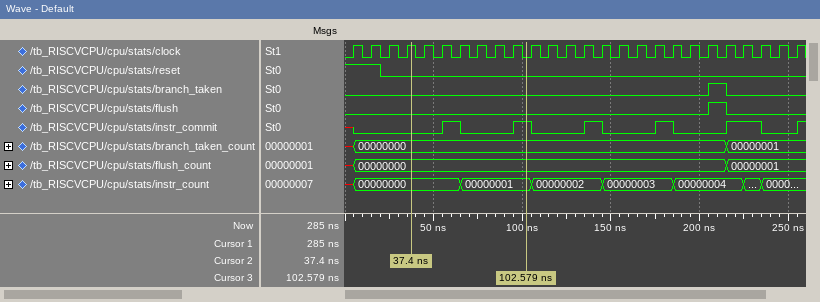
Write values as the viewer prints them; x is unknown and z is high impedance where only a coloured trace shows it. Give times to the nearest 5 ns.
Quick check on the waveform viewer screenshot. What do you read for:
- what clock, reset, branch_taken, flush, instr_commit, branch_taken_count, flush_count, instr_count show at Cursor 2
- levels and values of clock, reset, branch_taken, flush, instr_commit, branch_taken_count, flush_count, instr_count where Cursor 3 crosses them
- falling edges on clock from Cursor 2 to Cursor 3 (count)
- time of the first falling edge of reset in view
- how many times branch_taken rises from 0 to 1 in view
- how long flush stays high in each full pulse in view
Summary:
clock=1, reset=0, branch_taken=0, flush=0, instr_commit=0, branch_taken_count=00000000, flush_count=00000000, instr_count=00000000
clock=0, reset=0, branch_taken=0, flush=0, instr_commit=1, branch_taken_count=00000000, flush_count=00000000, instr_count=00000001
7
20 ns
1
10 ns
